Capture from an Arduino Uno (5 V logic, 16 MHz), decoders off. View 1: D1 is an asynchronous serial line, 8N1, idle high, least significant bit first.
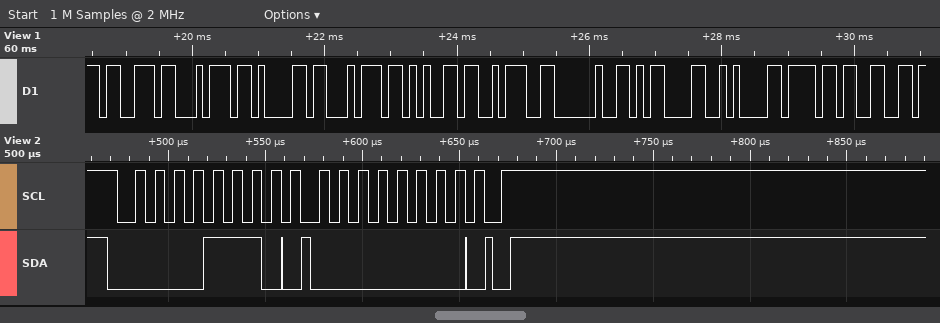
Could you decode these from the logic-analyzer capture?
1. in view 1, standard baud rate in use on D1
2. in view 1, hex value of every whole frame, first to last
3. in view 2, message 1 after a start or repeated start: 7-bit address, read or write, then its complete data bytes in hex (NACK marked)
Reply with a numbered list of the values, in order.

1. 9600 baud
2. 73 74 61 74 65 3A 20 0D 0A 6F 66
3. 0x07 write: 00
